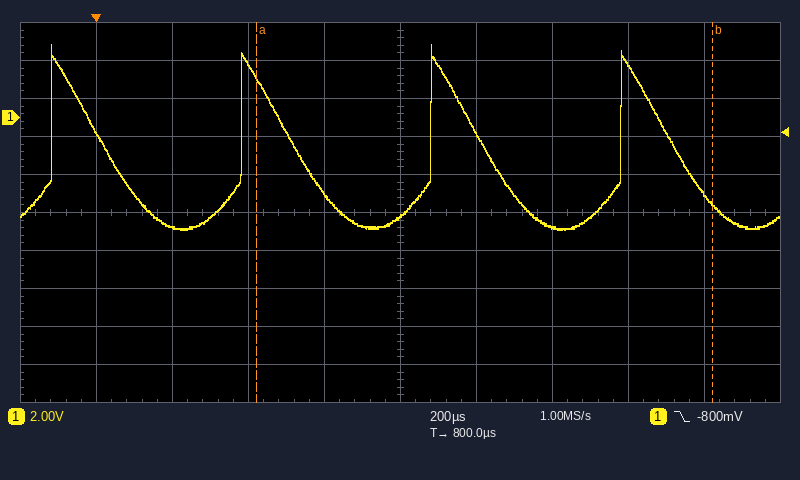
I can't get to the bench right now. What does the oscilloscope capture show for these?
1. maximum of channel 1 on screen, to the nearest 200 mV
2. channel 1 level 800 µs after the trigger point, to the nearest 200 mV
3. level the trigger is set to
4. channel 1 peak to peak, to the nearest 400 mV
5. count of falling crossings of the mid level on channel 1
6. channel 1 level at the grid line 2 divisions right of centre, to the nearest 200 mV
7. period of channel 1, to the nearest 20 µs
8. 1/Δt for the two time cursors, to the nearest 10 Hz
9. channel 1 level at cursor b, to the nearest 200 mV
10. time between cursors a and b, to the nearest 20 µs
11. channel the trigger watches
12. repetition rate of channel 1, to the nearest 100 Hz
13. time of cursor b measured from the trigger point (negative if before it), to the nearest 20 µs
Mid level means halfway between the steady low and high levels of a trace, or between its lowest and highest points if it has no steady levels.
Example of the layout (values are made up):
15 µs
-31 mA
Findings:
3.8 V
-5.2 V
-800 mV
9.6 V
4
-5.8 V
500 µs
830 Hz
-4.6 V
1.20 ms
channel 1
2.0 kHz
+1.62 ms
